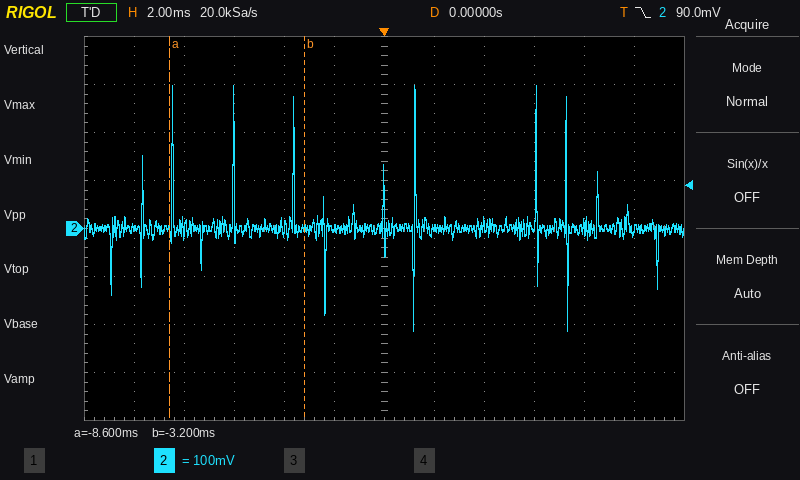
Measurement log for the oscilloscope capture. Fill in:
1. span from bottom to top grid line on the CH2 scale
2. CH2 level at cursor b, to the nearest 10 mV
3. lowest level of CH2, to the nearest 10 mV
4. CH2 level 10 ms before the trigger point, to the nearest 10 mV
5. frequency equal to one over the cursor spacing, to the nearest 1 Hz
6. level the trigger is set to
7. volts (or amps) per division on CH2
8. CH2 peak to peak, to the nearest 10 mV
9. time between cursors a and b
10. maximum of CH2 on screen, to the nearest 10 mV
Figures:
800 mV
0 mV
-210 mV
0 mV
185 Hz
90.0 mV
100 mV
510 mV
5.4 ms
300 mV
